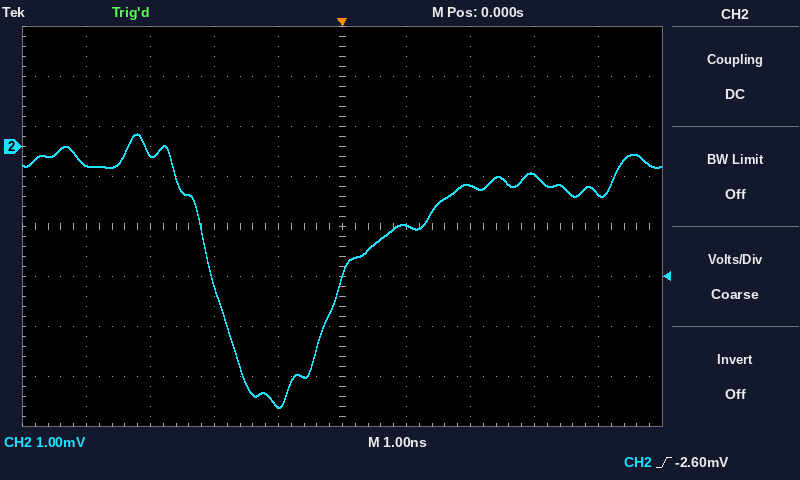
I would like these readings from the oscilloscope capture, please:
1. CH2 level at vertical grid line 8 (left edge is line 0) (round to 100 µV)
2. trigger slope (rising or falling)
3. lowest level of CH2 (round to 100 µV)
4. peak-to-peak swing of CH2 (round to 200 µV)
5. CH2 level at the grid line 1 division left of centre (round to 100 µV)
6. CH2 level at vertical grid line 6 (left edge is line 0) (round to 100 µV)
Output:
-600 µV
rising
-5.2 mV
5.4 mV
-5.2 mV
-1.6 mV
